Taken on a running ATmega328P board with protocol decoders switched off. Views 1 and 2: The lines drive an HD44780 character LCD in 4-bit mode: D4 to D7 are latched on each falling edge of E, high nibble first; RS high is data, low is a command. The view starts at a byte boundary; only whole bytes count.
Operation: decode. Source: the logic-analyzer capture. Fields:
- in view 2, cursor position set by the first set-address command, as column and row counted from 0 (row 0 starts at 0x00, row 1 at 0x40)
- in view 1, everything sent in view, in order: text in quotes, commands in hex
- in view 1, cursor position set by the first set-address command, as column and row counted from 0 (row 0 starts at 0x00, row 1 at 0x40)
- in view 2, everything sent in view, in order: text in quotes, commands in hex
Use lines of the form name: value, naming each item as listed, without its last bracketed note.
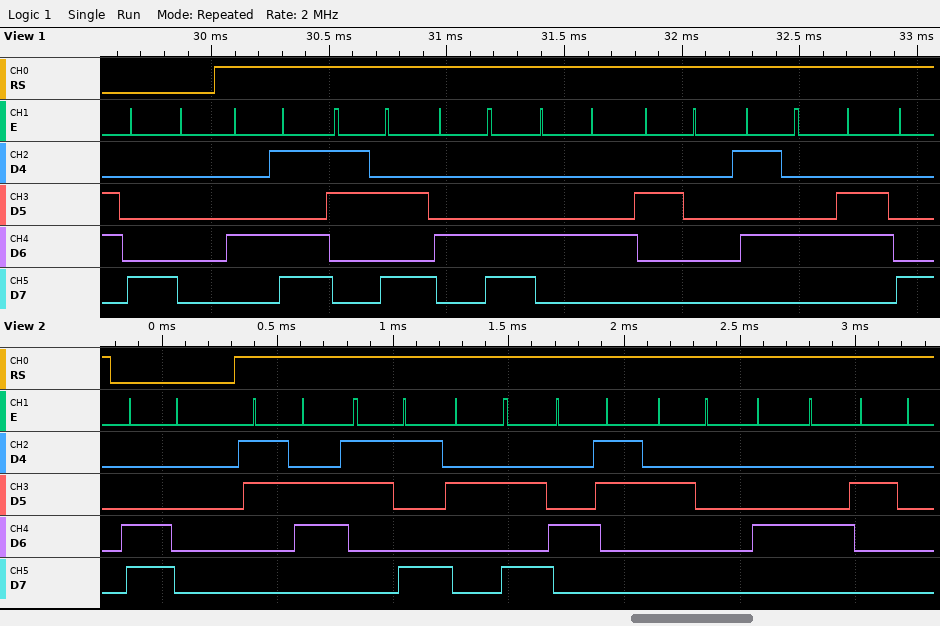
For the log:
in view 2, cursor position set by the first set-address command, as column and row counted from 0: column 0, row 1
in view 1, everything sent in view, in order: text in quotes, commands in hex: 0x80 "M:LD Th"
in view 1, cursor position set by the first set-address command, as column and row counted from 0: column 0, row 0
in view 2, everything sent in view, in order: text in quotes, commands in hex: 0xC0 "69*C D "
